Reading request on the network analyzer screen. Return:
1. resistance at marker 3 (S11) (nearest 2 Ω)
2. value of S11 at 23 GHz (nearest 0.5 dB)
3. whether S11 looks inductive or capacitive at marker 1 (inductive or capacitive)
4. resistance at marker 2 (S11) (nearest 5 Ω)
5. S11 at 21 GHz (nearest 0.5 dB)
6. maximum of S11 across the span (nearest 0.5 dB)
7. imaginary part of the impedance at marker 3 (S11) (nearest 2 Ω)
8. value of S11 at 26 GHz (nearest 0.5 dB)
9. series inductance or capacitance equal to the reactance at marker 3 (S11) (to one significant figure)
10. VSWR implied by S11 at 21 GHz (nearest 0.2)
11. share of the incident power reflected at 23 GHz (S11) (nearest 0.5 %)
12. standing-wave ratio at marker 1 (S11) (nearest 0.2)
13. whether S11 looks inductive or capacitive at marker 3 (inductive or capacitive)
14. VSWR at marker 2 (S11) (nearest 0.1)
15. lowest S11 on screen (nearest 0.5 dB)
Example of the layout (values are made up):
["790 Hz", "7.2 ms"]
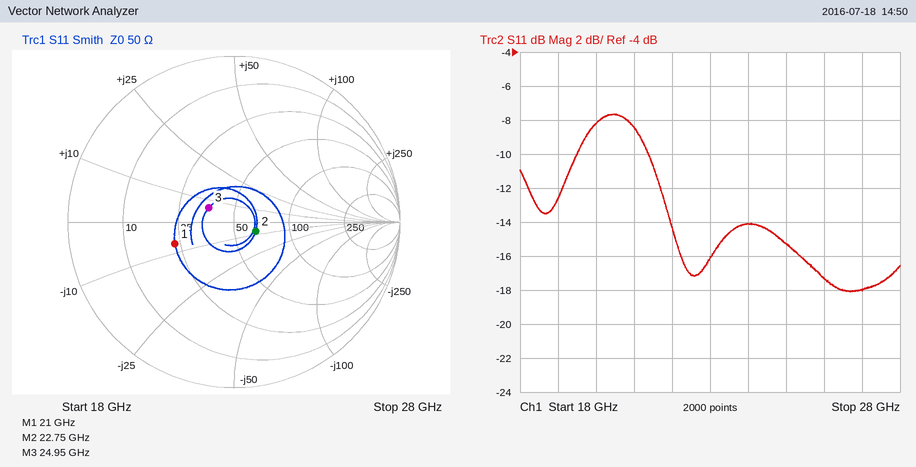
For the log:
["36 Ω", "-16.0 dB", "capacitive", "65 Ω", "-8.5 dB", "-7.5 dB", "+6 Ω", "-17.5 dB", "40 pH", "2.2", "2.5 %", "2.2", "inductive", "1.3", "-18.0 dB"]
